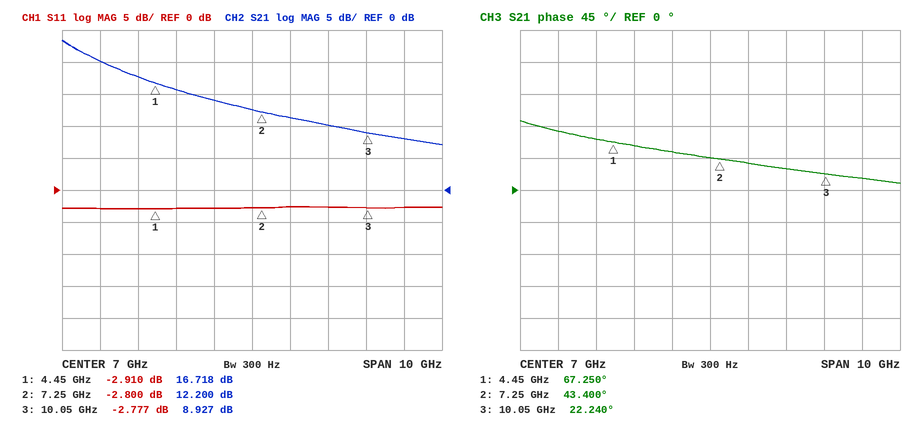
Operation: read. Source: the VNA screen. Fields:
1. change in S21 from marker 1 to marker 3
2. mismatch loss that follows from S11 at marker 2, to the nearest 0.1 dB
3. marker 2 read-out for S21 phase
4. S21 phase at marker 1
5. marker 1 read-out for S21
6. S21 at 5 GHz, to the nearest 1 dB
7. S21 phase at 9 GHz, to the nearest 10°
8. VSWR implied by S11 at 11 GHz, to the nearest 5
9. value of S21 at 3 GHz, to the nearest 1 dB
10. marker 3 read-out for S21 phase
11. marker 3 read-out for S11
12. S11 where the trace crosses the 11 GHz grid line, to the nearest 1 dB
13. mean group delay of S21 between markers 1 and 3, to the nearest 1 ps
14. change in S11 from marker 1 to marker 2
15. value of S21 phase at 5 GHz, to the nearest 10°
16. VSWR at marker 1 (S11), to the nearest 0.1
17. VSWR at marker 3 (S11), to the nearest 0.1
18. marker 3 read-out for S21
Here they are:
-7.791 dB
3.2 dB
43.400°
67.250°
16.718 dB
16 dB
30°
5
20 dB
22.240°
-2.777 dB
-3 dB
22 ps
0.110 dB
60°
6.0
6.3
8.927 dB
